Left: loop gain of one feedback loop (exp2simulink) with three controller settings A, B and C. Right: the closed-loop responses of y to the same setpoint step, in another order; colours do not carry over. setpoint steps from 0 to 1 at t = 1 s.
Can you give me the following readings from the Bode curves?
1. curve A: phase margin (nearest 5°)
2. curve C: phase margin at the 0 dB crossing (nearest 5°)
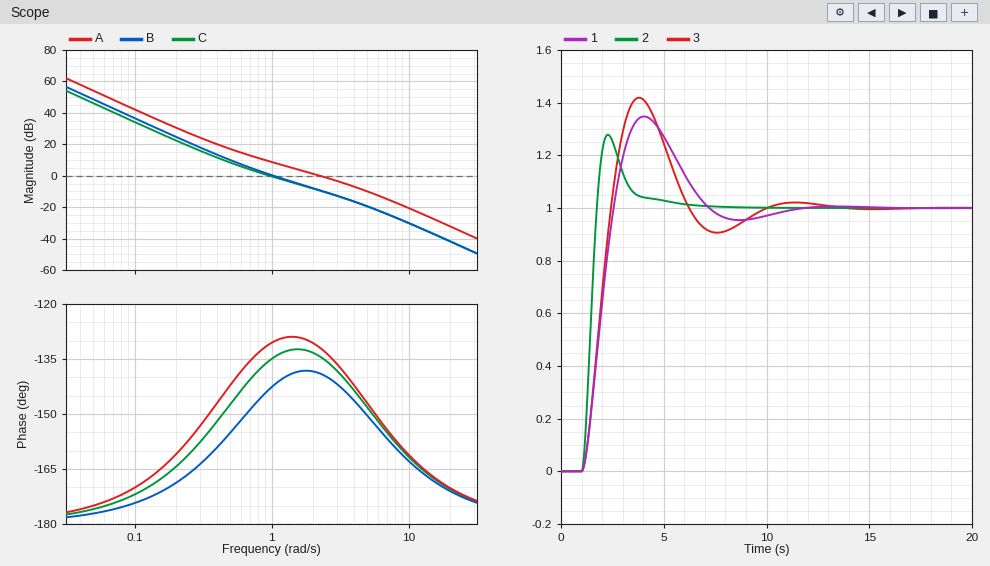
50°
45°
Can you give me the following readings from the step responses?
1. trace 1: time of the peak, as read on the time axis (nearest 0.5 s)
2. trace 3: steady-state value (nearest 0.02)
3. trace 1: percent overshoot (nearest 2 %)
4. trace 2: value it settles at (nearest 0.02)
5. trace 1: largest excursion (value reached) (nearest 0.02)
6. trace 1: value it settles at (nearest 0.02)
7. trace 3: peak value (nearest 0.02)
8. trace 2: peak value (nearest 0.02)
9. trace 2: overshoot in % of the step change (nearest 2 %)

4.0 s
1.00
34 %
1.00
1.34
1.00
1.42
1.28
28 %
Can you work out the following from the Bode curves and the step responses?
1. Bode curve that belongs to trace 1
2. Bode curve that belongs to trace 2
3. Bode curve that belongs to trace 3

C
A
B
